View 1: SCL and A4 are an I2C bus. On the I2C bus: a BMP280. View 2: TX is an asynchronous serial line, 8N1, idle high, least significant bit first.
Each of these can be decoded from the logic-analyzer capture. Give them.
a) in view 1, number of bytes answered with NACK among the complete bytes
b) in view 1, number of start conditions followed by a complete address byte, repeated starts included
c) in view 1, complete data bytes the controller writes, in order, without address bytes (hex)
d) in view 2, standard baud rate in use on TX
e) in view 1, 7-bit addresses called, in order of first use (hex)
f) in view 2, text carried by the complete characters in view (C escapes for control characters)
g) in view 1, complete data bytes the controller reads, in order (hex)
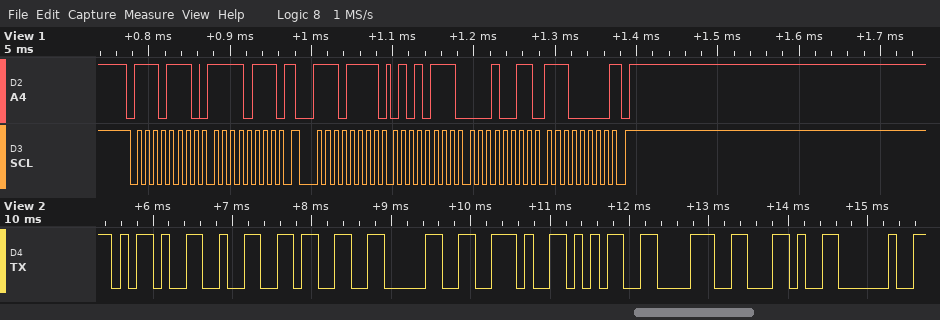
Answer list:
1
2
F7
9600 baud
0x77
"-230.58, "
57 13 E0
